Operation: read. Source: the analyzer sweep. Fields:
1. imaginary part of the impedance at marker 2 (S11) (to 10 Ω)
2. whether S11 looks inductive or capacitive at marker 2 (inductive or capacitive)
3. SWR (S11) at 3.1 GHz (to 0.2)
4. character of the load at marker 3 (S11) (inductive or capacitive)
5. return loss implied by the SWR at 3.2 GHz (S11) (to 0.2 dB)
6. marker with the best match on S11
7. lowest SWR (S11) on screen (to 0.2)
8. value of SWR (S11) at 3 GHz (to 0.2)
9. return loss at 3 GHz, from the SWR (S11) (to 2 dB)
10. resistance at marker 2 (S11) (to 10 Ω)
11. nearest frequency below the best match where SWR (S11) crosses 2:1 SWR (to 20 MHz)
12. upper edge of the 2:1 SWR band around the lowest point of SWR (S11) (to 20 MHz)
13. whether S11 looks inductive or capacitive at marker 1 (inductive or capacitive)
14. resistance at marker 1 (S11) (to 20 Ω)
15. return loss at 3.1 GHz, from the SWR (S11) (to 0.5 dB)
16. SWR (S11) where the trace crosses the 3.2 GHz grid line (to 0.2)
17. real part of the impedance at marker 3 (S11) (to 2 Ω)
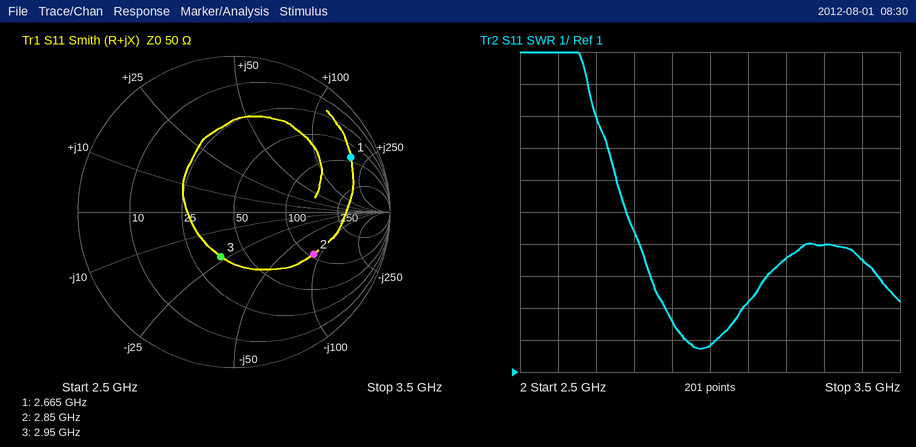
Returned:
-90 Ω
capacitive
3.2
capacitive
3.8 dB
marker 3
1.8
1.8
10 dB
110 Ω
2.94 GHz
3.02 GHz
inductive
80 Ω
5.5 dB
4.6
36 Ω
